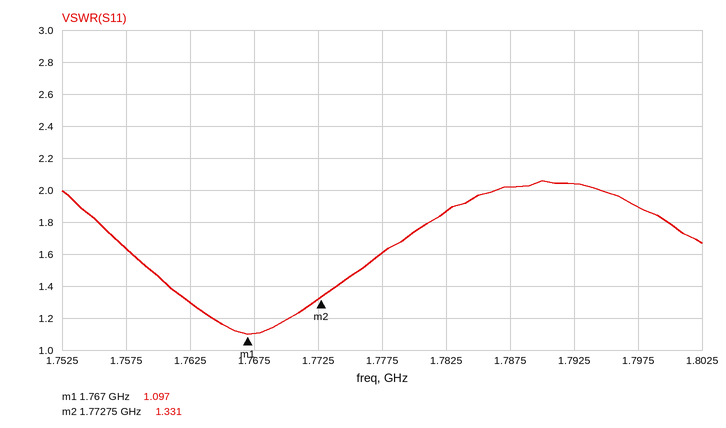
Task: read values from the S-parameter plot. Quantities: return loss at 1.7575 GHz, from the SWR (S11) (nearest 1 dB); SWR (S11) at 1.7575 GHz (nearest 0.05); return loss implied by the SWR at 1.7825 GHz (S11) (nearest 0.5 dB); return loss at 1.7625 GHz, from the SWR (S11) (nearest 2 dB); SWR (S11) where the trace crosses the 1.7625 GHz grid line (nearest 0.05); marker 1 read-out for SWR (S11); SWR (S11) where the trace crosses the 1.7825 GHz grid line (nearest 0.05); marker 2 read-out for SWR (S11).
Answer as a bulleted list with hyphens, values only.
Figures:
- 12 dB
- 1.65
- 10.5 dB
- 18 dB
- 1.30
- 1.097
- 1.85
- 1.331
